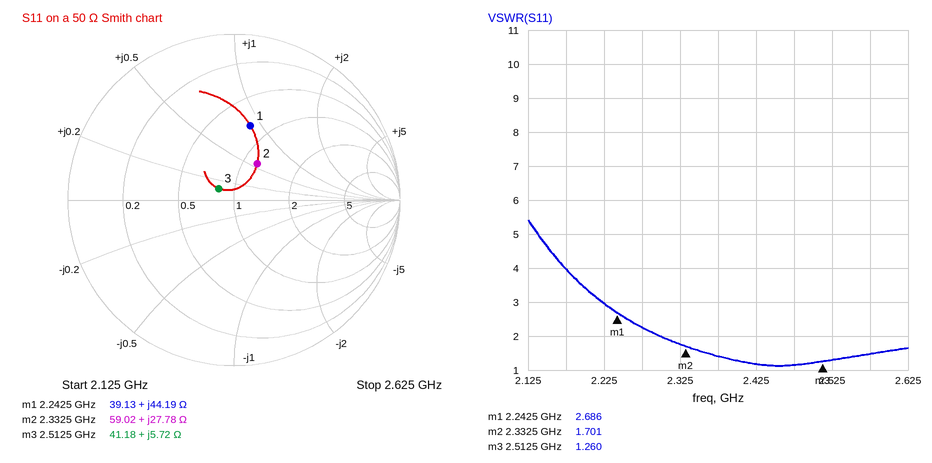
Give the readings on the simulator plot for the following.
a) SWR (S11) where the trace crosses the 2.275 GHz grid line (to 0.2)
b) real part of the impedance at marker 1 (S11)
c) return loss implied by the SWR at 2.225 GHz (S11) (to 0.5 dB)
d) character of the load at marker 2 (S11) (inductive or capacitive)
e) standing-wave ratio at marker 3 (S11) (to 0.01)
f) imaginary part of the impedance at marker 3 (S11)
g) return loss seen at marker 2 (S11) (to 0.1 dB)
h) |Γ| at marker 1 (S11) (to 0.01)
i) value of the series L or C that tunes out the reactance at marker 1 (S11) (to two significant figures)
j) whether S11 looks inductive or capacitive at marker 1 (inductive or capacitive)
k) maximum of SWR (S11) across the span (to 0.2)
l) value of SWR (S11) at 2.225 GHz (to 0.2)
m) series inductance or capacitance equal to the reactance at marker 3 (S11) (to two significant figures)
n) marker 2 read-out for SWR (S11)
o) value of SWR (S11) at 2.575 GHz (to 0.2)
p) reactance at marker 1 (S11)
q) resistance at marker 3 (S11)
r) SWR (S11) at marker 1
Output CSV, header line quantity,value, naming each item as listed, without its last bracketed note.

quantity,value
SWR (S11) where the trace crosses the 2.275 GHz grid line,2.2
real part of the impedance at marker 1,39.13 Ω
return loss implied by the SWR at 2.225 GHz (S11),6.0 dB
character of the load at marker 2 (S11),inductive
standing-wave ratio at marker 3 (S11),1.26
imaginary part of the impedance at marker 3,+5.72 Ω
return loss seen at marker 2 (S11),11.7 dB
|Γ| at marker 1 (S11),0.46
value of the series L or C that tunes out the reactance at marker 1 (S11),1.6 pF
whether S11 looks inductive or capacitive at marker 1,inductive
maximum of SWR (S11) across the span,5.4
value of SWR (S11) at 2.225 GHz,3.0
series inductance or capacitance equal to the reactance at marker 3 (S11),360 pH
marker 2 read-out for SWR,1.701
value of SWR (S11) at 2.575 GHz,1.4
reactance at marker 1,+44.19 Ω
resistance at marker 3,41.18 Ω
SWR (S11) at marker 1,2.686
